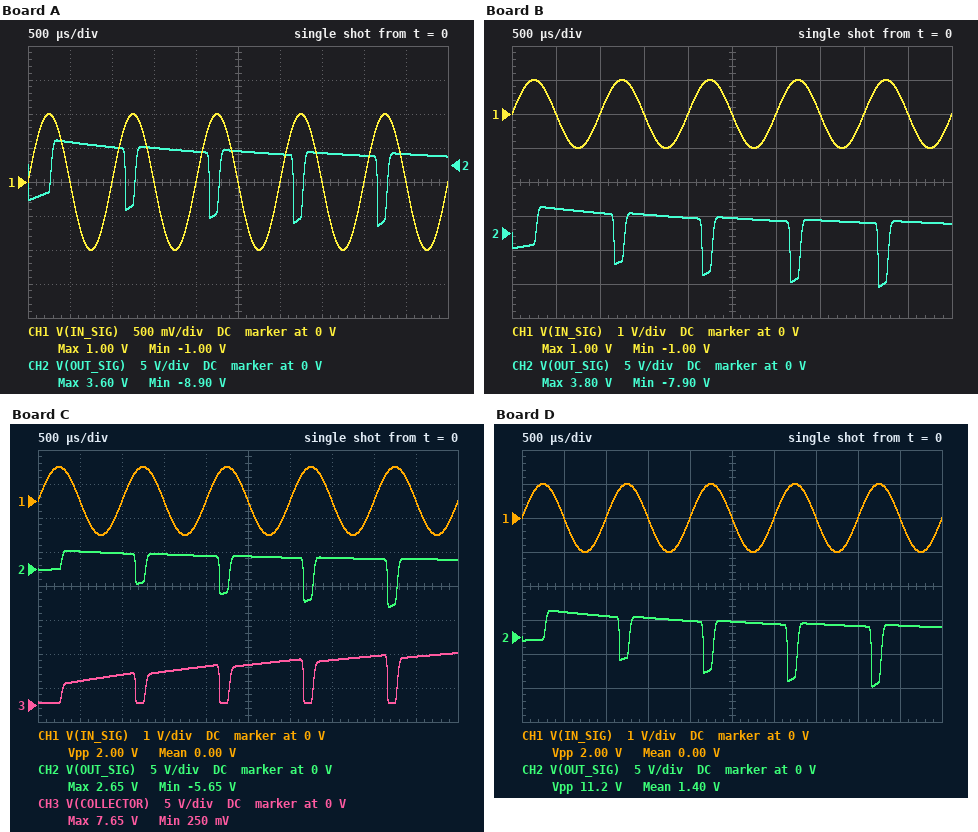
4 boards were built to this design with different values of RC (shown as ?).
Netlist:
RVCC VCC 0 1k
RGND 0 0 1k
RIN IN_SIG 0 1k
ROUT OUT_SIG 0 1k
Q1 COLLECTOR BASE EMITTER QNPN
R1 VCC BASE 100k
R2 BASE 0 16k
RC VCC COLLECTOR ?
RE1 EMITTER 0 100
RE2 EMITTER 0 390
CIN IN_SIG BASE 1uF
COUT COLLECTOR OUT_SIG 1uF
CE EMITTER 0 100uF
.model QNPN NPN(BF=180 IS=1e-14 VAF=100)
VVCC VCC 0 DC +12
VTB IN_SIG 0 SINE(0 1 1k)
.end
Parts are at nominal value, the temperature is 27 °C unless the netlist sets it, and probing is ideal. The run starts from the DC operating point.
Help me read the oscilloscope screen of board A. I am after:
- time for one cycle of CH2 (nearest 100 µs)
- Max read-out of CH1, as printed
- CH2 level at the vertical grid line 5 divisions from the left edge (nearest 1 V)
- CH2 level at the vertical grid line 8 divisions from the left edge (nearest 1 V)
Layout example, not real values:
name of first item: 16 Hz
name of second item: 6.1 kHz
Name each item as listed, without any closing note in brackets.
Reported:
time for one cycle of CH2: 1.0 ms
Max read-out of CH1, as printed: 1.00 V
CH2 level at the vertical grid line 5 divisions from the left edge: 2 V
CH2 level at the vertical grid line 8 divisions from the left edge: 1 V
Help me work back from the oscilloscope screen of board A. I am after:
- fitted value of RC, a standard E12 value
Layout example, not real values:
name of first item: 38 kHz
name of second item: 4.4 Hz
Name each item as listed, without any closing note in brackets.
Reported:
fitted value of RC, a standard E12 value: 1 kΩ
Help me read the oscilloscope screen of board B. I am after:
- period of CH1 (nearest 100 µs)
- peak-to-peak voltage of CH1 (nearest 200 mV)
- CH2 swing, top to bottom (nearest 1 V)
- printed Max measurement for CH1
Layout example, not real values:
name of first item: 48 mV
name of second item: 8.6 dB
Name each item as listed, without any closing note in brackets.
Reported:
period of CH1: 1.0 ms
peak-to-peak voltage of CH1: 2.0 V
CH2 swing, top to bottom: 12 V
printed Max measurement for CH1: 1.00 V
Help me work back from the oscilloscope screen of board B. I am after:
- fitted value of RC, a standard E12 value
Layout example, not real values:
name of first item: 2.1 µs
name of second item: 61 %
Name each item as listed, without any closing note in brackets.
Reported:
fitted value of RC, a standard E12 value: 1.5 kΩ
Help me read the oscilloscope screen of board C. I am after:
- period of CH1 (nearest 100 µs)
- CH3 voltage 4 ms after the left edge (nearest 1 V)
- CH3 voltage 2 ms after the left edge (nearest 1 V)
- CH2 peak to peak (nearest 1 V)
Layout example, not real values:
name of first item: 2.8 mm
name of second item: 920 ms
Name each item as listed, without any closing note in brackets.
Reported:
period of CH1: 1.0 ms
CH3 voltage 4 ms after the left edge: 7 V
CH3 voltage 2 ms after the left edge: 6 V
CH2 peak to peak: 8 V
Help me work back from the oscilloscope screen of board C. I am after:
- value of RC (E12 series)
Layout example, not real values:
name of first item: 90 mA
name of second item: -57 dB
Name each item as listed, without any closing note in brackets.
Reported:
value of RC: 3.3 kΩ
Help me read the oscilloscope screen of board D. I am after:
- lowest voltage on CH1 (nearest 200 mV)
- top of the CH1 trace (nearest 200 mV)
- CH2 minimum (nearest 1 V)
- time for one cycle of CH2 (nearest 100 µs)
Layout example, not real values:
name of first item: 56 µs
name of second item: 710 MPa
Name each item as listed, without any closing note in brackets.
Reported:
lowest voltage on CH1: -1.0 V
top of the CH1 trace: 1.0 V
CH2 minimum: -7 V
time for one cycle of CH2: 1.0 ms
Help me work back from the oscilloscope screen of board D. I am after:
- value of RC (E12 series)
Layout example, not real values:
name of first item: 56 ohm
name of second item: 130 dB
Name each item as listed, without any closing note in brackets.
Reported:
value of RC: 1.8 kΩ
